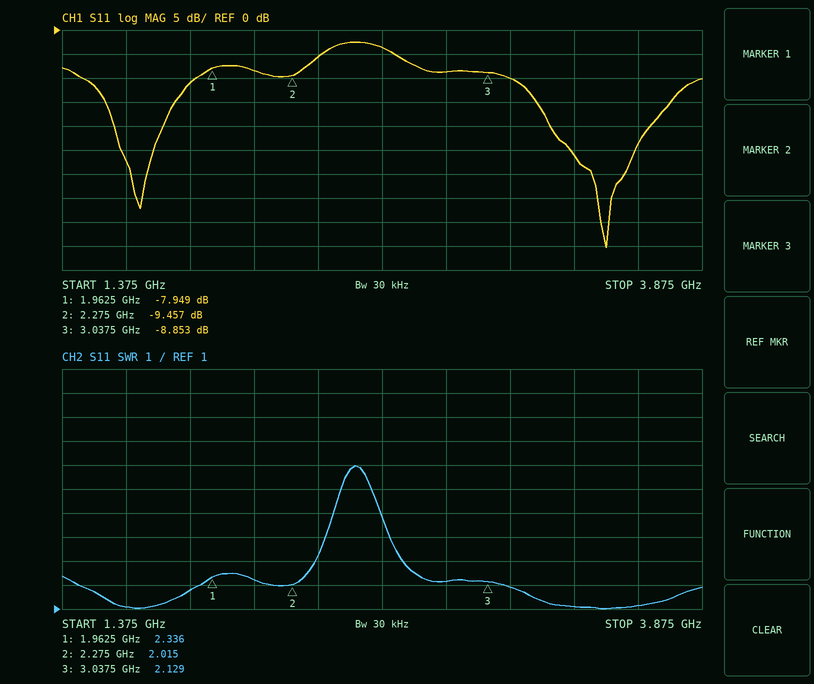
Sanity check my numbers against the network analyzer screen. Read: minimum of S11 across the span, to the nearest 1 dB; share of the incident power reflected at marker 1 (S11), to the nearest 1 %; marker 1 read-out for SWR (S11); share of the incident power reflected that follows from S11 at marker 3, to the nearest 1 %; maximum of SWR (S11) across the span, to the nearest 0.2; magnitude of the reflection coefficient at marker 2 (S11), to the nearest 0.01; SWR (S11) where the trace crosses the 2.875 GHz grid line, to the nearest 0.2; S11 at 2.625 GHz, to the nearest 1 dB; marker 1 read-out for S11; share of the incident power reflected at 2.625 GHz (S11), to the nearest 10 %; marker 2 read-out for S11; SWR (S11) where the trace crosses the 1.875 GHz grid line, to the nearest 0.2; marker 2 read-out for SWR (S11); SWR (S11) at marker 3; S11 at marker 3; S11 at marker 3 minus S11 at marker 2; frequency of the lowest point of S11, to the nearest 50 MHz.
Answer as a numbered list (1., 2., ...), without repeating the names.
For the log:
1. -45 dB
2. 16 %
3. 2.336
4. 13 %
5. 7.0
6. 0.34
7. 2.2
8. -4 dB
9. -7.949 dB
10. 40 %
11. -9.457 dB
12. 1.8
13. 2.015
14. 2.129
15. -8.853 dB
16. 0.604 dB
17. 3.50 GHz
